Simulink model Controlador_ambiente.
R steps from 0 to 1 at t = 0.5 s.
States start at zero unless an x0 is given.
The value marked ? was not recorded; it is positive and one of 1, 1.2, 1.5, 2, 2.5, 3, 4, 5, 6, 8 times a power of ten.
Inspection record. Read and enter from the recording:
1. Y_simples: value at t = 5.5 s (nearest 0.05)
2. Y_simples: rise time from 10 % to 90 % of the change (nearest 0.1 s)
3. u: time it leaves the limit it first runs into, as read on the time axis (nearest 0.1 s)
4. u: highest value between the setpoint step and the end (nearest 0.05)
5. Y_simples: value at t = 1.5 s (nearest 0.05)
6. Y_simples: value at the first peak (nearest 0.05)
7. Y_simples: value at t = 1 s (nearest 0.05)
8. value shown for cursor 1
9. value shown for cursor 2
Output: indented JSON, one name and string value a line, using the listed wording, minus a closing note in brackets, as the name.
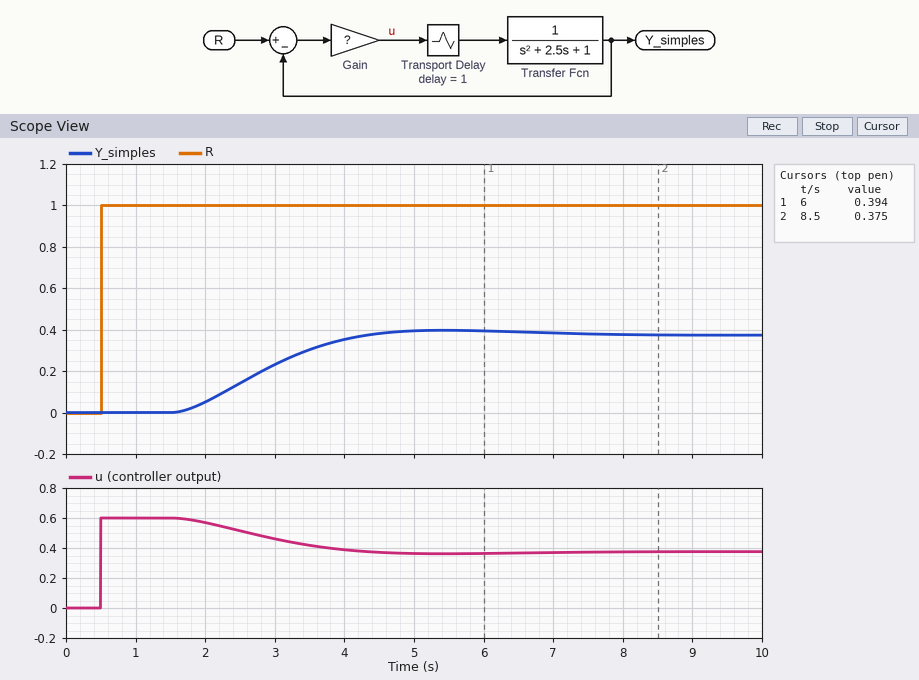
{
  "Y_simples: value at t = 5.5 s": "0.40",
  "Y_simples: rise time from 10 % to 90 % of the change": "1.9 s",
  "u: time it leaves the limit it first runs into, as read on the time axis": "1.7 s",
  "u: highest value between the setpoint step and the end": "0.60",
  "Y_simples: value at t = 1.5 s": "0.00",
  "Y_simples: value at the first peak": "0.40",
  "Y_simples: value at t = 1 s": "0.00",
  "value shown for cursor 1": "0.394",
  "value shown for cursor 2": "0.375"
}
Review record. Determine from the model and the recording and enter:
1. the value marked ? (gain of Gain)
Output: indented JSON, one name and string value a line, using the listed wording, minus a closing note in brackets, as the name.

{
  "the value marked ?": "0.6"
}
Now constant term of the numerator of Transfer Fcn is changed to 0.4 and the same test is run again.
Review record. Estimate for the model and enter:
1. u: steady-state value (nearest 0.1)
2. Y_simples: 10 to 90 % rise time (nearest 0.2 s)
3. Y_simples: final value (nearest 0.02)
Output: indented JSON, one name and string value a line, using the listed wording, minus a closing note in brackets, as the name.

{
  "u: steady-state value": "0.5",
  "Y_simples: 10 to 90 % rise time": "3.0 s",
  "Y_simples: final value": "0.20"
}
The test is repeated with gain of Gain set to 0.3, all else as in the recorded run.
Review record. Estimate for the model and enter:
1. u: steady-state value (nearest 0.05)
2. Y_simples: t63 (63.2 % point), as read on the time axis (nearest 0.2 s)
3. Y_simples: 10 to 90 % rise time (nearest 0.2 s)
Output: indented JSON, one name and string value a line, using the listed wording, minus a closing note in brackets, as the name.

{
  "u: steady-state value": "0.25",
  "Y_simples: t63 (63.2 % point), as read on the time axis": "3.4 s",
  "Y_simples: 10 to 90 % rise time": "2.8 s"
}
